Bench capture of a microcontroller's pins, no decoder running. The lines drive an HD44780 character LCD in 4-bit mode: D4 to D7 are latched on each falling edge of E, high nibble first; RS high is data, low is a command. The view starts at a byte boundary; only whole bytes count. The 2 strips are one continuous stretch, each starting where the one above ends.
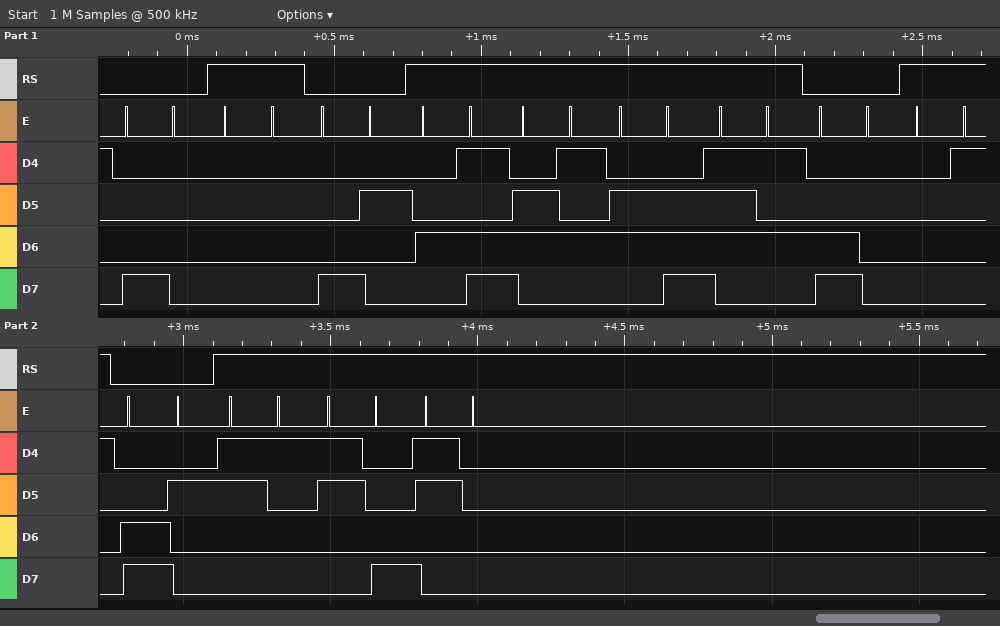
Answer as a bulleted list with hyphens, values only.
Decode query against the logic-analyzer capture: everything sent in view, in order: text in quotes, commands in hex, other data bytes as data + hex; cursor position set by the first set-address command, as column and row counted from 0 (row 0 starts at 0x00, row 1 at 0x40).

- 0x80 data 00 0x82 "Menu" 0xC0 data 01 0xC2 "180"
- column 0, row 0
